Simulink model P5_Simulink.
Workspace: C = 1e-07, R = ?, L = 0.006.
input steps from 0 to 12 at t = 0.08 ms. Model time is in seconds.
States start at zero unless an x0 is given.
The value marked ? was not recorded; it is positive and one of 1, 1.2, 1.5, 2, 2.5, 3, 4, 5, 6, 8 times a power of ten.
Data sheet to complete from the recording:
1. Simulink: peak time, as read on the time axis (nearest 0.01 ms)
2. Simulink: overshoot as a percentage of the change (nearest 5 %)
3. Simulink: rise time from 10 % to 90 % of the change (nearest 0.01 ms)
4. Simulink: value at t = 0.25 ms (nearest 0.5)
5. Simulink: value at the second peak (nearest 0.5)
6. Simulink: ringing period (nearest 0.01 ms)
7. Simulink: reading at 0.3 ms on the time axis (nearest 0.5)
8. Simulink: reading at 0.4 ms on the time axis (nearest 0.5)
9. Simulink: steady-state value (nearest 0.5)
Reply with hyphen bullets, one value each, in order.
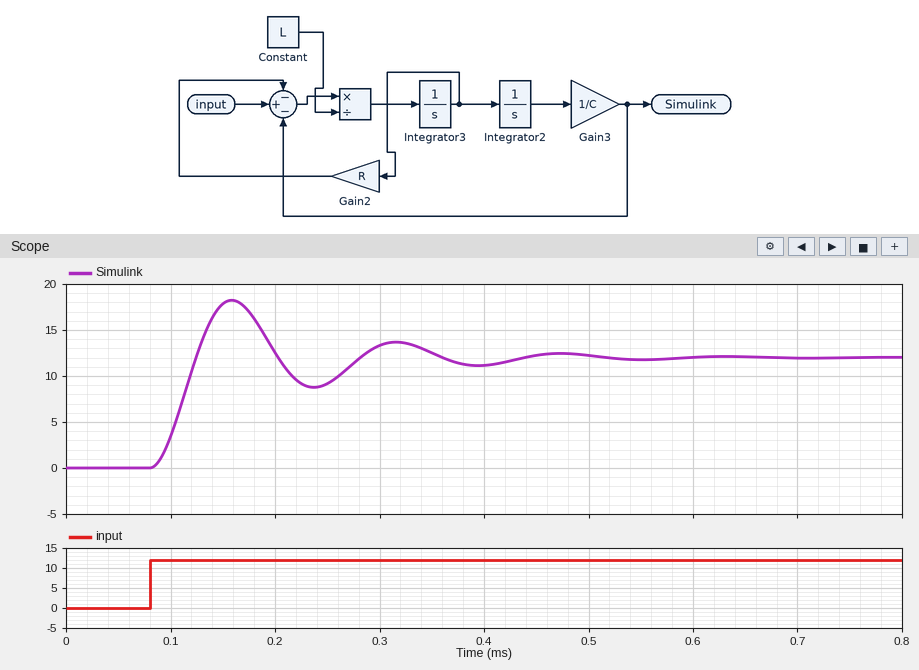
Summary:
- 0.16 ms
- 50 %
- 0.03 ms
- 9.0
- 13.5
- 0.16 ms
- 13.5
- 11.0
- 12.0
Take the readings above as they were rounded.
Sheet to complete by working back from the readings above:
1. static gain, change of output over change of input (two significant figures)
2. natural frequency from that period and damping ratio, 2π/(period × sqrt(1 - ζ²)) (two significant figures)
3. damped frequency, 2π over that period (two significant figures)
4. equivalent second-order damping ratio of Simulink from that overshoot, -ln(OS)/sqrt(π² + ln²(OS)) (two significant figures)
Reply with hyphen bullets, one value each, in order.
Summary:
- 1.0
- 40 rad/ms
- 39 rad/ms
- 0.22
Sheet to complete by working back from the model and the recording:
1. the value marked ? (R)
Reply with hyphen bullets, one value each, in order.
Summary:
- 100
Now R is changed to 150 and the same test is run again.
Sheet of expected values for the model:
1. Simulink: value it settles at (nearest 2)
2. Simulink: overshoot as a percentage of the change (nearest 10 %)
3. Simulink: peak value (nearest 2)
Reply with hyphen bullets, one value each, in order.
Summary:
- 12
- 40 %
- 16
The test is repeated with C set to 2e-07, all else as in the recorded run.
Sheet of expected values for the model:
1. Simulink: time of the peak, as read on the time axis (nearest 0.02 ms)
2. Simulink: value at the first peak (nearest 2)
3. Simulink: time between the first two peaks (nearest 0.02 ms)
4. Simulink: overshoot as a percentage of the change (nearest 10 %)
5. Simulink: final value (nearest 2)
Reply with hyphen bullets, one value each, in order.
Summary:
- 0.20 ms
- 16
- 0.22 ms
- 40 %
- 12
